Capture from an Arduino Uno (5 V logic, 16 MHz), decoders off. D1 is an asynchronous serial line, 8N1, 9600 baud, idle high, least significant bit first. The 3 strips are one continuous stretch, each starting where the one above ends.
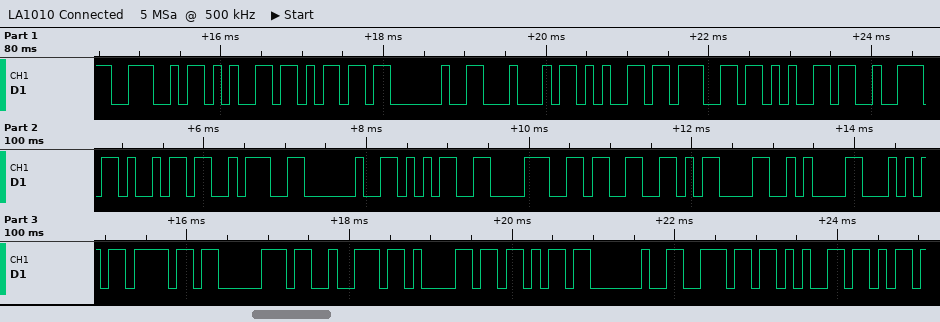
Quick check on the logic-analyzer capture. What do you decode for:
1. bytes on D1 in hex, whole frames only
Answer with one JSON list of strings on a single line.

["0x4E 0x65 0x6D 0x20 0x44 0x65 0x67 0x65 0x72 0x69 0x3A 0x20 0x35 0x38 0x33 0x0D 0x0A 0x54 0x6F 0x70 0x72 0x61 0x6B 0x20 0x6E 0x65"]
